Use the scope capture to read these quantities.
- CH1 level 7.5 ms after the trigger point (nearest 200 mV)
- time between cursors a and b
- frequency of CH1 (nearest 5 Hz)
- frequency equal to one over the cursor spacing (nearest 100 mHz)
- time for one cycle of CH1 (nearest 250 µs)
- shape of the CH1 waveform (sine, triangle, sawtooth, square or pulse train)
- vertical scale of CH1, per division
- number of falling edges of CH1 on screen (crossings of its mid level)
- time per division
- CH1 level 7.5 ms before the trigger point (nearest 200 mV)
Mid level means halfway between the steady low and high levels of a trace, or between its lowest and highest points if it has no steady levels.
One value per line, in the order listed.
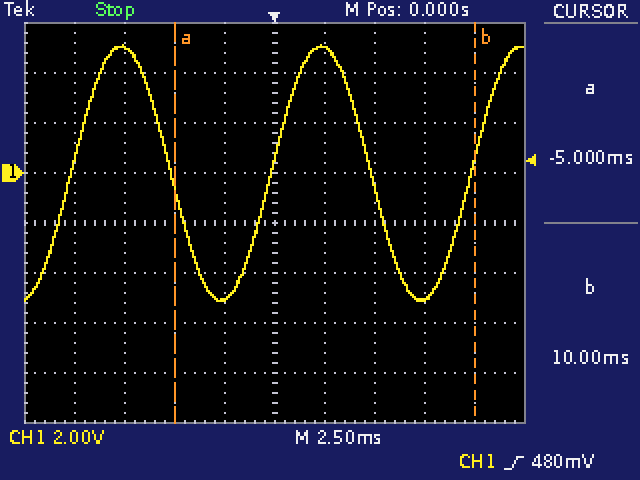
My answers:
-5.0 V
15.00 ms
100 Hz
66.7 Hz
10.00 ms
sine
2 V
2
2.5 ms
5.0 V
